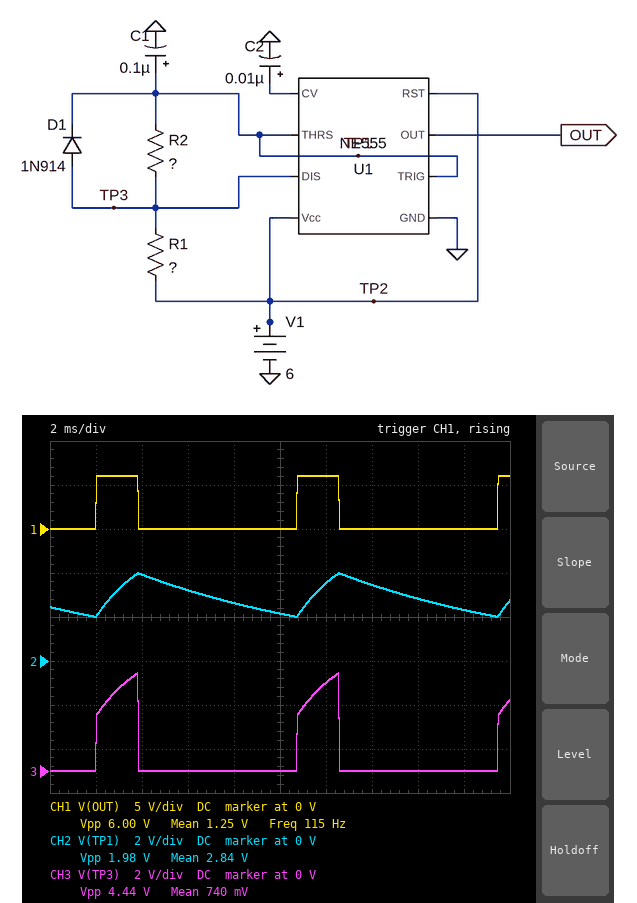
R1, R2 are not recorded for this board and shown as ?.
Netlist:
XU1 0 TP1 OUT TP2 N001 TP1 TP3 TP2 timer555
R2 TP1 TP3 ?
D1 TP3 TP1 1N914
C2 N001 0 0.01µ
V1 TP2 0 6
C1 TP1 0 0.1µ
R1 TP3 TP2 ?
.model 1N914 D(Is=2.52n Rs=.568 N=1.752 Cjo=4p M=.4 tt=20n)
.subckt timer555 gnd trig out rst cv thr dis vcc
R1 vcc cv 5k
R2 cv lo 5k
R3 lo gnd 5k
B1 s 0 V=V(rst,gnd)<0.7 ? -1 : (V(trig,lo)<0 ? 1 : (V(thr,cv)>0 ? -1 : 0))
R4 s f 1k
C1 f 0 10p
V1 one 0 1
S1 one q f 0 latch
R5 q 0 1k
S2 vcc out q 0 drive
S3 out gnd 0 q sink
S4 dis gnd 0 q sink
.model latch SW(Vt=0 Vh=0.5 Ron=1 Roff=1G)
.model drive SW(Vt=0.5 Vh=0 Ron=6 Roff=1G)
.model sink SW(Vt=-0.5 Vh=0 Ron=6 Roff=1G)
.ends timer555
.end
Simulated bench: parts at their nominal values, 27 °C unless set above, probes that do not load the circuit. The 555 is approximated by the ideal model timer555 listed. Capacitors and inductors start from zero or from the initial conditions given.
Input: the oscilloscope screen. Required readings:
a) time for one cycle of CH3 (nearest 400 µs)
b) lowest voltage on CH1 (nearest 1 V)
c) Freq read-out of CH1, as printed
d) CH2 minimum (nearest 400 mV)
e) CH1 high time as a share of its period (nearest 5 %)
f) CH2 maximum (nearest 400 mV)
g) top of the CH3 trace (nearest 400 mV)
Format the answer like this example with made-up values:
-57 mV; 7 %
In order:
8.8 ms; 0 V; 115 Hz; 2.0 V; 20 %; 4.0 V; 4.4 V
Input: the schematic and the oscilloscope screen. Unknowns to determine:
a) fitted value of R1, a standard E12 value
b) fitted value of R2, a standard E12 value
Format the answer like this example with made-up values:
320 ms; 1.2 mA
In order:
22 kΩ; 100 kΩ
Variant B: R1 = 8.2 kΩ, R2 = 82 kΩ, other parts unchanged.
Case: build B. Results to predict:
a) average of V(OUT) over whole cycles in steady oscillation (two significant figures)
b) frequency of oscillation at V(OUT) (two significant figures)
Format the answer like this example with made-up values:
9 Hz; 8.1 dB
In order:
660 mV; 160 Hz
